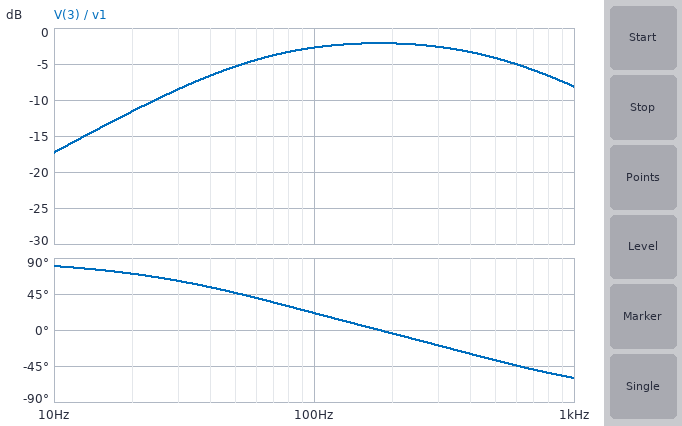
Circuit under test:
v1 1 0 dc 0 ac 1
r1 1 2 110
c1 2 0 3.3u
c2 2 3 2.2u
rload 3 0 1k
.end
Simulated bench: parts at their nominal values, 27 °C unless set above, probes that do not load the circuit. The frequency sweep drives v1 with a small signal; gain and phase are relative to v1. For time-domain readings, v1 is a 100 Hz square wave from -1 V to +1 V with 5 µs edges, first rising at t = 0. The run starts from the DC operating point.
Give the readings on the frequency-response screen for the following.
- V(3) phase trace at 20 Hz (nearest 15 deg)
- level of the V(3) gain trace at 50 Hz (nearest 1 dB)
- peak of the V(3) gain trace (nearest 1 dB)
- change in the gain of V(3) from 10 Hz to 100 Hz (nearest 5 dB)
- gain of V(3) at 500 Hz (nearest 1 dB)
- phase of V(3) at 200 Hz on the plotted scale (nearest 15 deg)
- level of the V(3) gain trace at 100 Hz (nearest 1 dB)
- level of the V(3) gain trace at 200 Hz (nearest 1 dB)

75 deg
-5 dB
-2 dB
15 dB
-4 dB
0 deg
-3 dB
-2 dB
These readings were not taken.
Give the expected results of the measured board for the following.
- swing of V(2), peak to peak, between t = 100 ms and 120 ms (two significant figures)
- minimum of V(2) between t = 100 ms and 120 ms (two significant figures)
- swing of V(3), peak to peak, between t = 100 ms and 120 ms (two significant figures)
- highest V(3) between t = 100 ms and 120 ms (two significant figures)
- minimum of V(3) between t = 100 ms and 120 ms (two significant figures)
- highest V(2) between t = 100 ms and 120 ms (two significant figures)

1.9 V
-970 mV
2.3 V
1.1 V
-1.1 V
970 mV
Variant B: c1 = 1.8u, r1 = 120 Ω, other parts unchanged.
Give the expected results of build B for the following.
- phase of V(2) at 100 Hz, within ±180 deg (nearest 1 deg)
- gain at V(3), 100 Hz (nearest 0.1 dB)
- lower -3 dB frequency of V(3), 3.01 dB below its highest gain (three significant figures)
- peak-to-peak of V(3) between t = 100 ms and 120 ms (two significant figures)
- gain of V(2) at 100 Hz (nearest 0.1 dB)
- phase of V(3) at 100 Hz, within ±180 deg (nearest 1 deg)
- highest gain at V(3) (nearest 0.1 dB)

-10 deg
-2.6 dB
55.9 Hz
2.5 V
-0.8 dB
26 deg
-1.7 dB
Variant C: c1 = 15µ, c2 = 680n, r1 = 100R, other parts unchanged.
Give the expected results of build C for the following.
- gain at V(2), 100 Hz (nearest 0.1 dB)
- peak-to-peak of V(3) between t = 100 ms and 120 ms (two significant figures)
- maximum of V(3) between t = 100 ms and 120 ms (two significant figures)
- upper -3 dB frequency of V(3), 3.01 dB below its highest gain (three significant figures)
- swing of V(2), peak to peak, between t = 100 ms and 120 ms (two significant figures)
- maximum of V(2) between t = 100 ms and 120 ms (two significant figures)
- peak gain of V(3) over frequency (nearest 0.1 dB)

-3.0 dB
860 mV
430 mV
411 Hz
1.8 V
920 mV
-10.4 dB
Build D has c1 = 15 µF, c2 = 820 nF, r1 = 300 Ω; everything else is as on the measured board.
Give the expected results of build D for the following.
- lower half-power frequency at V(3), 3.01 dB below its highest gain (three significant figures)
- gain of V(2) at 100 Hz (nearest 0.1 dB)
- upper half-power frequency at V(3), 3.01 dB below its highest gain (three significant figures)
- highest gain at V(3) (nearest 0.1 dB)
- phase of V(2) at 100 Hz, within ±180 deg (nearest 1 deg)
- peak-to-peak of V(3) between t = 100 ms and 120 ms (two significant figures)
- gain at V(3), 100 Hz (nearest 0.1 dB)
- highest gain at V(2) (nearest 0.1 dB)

25.8 Hz
-9.9 dB
266 Hz
-16.6 dB
-70 deg
340 mV
-16.7 dB
0 dB
